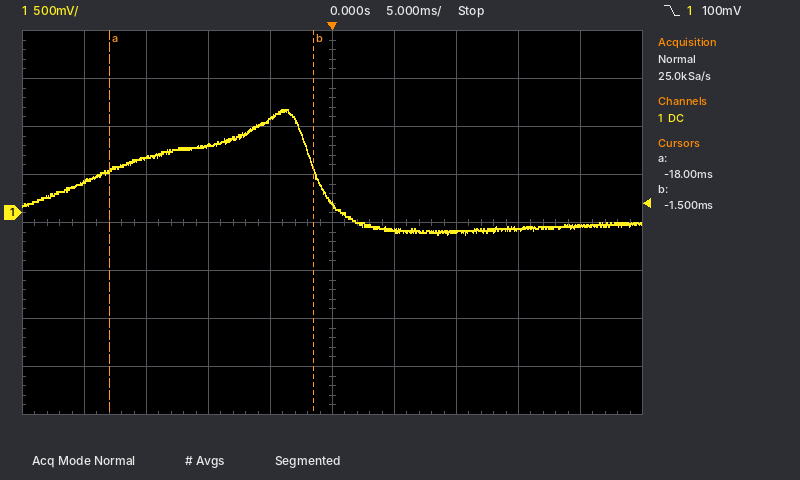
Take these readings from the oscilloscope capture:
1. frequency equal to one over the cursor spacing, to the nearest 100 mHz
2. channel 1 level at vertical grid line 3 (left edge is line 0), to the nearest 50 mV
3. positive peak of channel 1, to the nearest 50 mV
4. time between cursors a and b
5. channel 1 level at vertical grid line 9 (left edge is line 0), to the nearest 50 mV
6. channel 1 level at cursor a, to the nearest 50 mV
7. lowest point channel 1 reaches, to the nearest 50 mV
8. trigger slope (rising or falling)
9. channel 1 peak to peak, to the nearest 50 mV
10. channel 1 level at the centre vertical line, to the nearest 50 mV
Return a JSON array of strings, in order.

["60.6 Hz", "700 mV", "1.10 V", "16.5 ms", "-150 mV", "450 mV", "-200 mV", "falling", "1.30 V", "100 mV"]
